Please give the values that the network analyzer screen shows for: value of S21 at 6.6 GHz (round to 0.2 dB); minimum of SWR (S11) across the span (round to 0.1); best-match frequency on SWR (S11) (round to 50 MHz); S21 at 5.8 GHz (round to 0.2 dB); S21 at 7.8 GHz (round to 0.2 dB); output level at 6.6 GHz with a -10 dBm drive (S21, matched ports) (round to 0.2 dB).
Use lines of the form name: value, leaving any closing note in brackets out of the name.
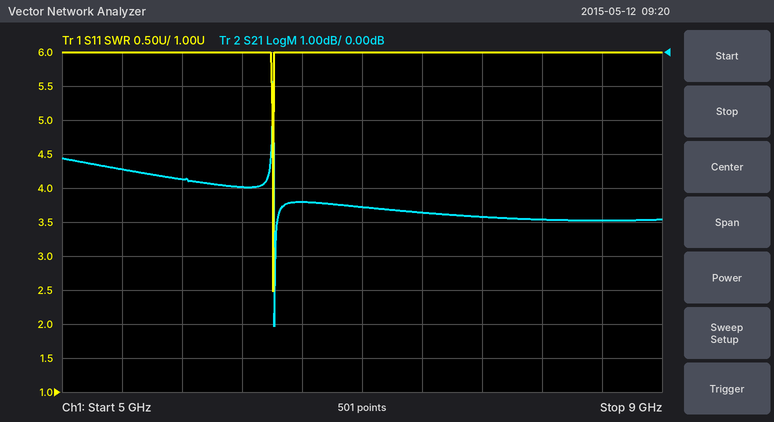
value of S21 at 6.6 GHz: -4.4 dB
minimum of SWR (S11) across the span: 2.5
best-match frequency on SWR (S11): 6.40 GHz
S21 at 5.8 GHz: -3.8 dB
S21 at 7.8 GHz: -4.8 dB
output level at 6.6 GHz with a -10 dBm drive (S21, matched ports): -14.4 dBm
